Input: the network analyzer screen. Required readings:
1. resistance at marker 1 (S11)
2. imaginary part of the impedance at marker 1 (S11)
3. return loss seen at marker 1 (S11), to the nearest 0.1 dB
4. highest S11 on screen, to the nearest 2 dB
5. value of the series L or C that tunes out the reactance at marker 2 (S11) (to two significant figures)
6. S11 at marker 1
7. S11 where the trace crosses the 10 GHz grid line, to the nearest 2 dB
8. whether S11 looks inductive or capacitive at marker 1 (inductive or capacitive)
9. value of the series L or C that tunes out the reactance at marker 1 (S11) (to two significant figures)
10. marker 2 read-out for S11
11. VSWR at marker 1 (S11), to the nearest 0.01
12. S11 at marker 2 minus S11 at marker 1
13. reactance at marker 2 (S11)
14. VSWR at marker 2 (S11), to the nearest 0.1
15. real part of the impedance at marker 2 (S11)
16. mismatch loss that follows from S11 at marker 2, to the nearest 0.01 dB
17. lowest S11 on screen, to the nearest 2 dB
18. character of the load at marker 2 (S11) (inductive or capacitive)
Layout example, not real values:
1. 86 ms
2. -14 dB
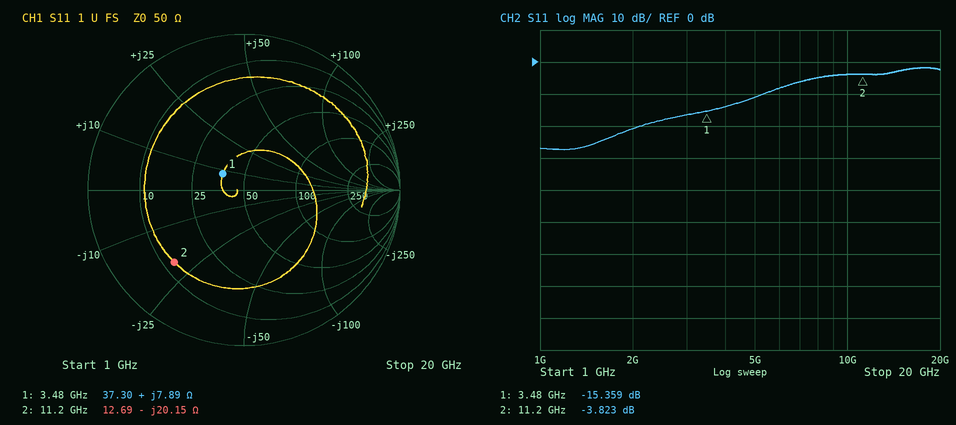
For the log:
1. 37.30 Ω
2. +7.89 Ω
3. 15.4 dB
4. -2 dB
5. 290 pH
6. -15.359 dB
7. -4 dB
8. inductive
9. 5.8 pF
10. -3.823 dB
11. 1.41
12. 11.536 dB
13. -20.15 Ω
14. 4.6
15. 12.69 Ω
16. 2.33 dB
17. -28 dB
18. capacitive
